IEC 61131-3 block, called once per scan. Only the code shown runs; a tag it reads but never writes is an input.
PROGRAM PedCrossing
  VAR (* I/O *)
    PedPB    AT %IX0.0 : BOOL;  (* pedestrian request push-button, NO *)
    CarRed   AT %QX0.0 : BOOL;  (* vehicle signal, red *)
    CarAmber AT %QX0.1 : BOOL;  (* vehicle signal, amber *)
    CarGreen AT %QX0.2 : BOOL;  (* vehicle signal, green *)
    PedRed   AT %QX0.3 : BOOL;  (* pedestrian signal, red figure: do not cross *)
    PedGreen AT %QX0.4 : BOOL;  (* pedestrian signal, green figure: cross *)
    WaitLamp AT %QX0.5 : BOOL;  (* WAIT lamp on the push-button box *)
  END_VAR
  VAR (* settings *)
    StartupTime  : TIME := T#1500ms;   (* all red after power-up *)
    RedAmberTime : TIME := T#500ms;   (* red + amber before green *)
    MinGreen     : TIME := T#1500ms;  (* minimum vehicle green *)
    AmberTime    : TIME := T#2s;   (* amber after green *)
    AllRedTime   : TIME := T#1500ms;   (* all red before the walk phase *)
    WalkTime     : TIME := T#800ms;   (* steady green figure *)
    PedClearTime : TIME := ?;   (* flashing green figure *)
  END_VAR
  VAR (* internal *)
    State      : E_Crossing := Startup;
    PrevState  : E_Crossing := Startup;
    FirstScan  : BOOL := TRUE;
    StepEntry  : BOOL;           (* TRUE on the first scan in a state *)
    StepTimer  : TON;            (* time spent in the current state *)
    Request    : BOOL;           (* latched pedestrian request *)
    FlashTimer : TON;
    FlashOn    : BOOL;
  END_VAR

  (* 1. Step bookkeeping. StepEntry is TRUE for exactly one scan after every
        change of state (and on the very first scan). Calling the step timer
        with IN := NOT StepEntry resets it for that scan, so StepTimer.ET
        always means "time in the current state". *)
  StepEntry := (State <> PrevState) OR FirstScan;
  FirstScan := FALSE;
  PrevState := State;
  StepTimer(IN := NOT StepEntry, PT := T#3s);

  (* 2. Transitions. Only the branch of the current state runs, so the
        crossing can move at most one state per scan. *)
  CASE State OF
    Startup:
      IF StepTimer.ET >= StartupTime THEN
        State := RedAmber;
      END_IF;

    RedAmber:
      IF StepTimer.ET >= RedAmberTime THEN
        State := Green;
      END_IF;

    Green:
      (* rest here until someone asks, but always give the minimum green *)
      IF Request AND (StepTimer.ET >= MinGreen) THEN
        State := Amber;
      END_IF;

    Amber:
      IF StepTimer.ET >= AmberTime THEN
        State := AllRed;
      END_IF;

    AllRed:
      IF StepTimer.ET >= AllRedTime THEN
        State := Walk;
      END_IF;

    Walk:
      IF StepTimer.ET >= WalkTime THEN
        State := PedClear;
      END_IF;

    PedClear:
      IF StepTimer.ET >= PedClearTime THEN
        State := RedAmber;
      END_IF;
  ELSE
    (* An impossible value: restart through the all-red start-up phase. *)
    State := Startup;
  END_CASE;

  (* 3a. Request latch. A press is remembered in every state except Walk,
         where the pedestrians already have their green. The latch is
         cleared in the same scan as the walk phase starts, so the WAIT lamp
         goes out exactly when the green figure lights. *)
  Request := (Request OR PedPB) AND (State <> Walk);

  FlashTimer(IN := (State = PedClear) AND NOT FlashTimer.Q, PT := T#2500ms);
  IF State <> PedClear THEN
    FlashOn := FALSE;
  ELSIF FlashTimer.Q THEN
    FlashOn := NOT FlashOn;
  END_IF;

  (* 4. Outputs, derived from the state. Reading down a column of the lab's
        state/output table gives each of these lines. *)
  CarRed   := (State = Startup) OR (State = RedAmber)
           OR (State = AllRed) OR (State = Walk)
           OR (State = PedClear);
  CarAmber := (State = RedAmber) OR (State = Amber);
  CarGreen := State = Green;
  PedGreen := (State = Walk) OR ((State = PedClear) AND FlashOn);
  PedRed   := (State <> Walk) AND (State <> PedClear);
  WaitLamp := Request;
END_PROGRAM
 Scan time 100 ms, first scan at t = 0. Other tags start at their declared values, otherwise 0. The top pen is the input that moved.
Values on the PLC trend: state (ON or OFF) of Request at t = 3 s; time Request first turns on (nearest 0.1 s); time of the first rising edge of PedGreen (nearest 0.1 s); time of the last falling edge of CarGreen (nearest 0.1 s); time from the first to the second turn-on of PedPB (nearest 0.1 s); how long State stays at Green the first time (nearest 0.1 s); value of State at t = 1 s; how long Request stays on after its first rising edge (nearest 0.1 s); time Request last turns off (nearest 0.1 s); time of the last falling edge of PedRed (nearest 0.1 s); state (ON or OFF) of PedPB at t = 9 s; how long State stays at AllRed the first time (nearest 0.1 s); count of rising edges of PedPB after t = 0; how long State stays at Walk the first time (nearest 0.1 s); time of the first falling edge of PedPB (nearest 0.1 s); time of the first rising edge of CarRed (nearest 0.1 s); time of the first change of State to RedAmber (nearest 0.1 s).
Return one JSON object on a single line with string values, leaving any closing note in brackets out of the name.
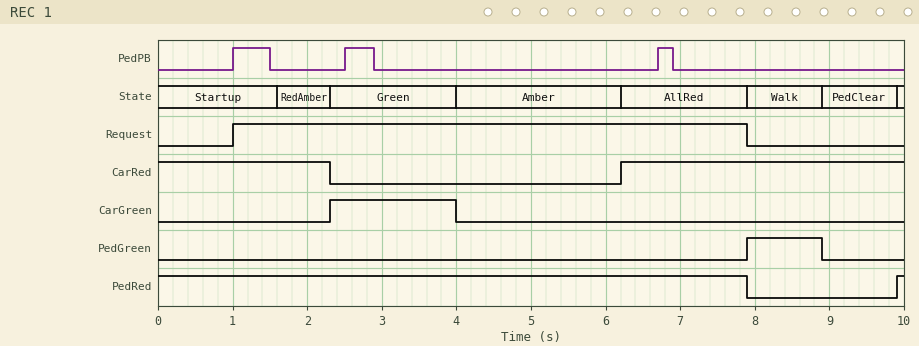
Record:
{"state (ON or OFF) of Request at t = 3 s": "ON", "time Request first turns on": "1.0 s", "time of the first rising edge of PedGreen": "7.9 s", "time of the last falling edge of CarGreen": "4.0 s", "time from the first to the second turn-on of PedPB": "1.5 s", "how long State stays at Green the first time": "1.7 s", "value of State at t = 1 s": "Startup", "how long Request stays on after its first rising edge": "6.9 s", "time Request last turns off": "7.9 s", "time of the last falling edge of PedRed": "7.9 s", "state (ON or OFF) of PedPB at t = 9 s": "OFF", "how long State stays at AllRed the first time": "1.7 s", "count of rising edges of PedPB after t = 0": "3", "how long State stays at Walk the first time": "1.0 s", "time of the first falling edge of PedPB": "1.5 s", "time of the first rising edge of CarRed": "6.2 s", "time of the first change of State to RedAmber": "1.6 s"}
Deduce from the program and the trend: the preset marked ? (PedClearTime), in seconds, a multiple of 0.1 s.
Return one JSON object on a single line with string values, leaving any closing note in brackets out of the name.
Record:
{"the preset marked ? (PedClearTime), in seconds, a multiple of 0.1 s": "0.8 s"}
